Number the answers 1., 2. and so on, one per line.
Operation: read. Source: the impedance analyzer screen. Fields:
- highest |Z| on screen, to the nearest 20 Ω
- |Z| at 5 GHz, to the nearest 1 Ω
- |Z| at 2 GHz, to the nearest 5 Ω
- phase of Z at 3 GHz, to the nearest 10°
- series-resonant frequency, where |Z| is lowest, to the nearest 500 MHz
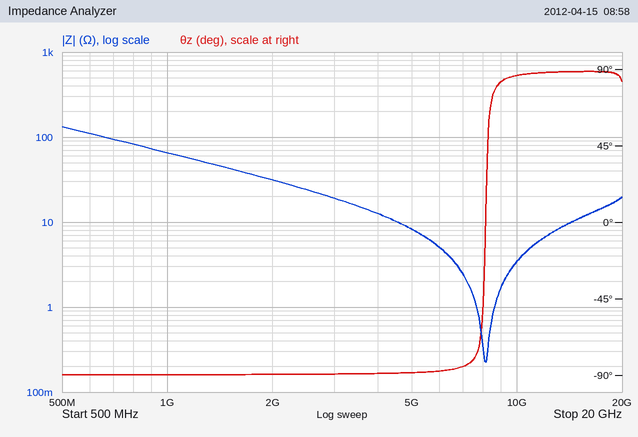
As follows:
1. 140 Ω
2. 8 Ω
3. 30 Ω
4. -90°
5. 8.0 GHz
